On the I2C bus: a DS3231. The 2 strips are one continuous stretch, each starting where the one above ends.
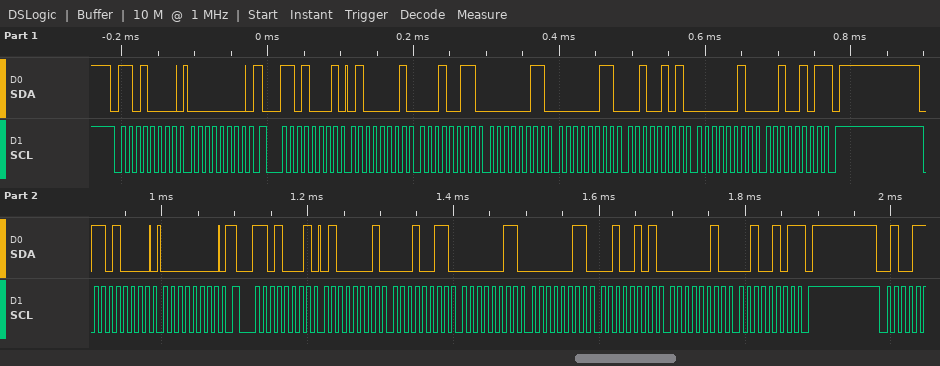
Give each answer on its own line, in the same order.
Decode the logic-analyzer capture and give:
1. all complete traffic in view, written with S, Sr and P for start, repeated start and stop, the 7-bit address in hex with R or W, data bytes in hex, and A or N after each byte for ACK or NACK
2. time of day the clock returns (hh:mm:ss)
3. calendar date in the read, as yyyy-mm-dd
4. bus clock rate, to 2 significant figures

S 68W A 00 A Sr 68R A 41 A 13 A 03 A 03 A 25 A 02 A 25 N P S 68W A 00 A Sr 68R A 41 A 13 A 03 A 03 A 25 A 02 A 25 N P
03:13:41
2025-02-25
100 kHz
